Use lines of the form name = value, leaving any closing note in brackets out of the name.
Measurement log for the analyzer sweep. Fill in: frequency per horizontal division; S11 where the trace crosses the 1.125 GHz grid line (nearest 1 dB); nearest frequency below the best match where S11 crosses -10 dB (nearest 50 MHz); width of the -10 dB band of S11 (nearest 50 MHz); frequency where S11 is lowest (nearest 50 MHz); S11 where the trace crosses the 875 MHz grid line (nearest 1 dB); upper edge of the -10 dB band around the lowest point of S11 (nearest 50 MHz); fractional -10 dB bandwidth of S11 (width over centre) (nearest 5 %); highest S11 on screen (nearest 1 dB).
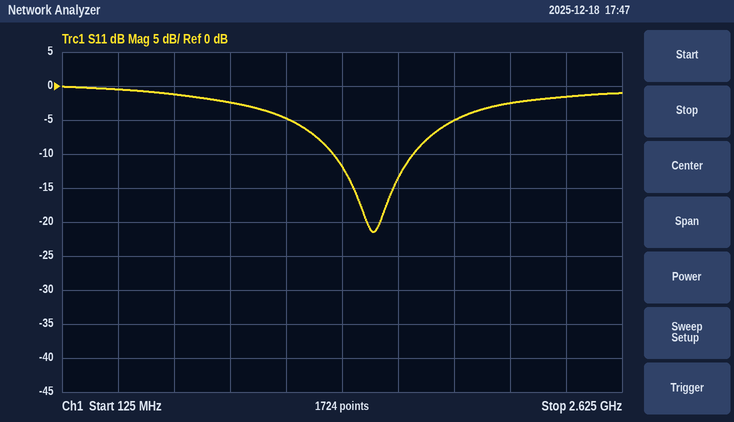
frequency per horizontal division = 250 MHz
S11 where the trace crosses the 1.125 GHz grid line = -5 dB
nearest frequency below the best match where S11 crosses -10 dB = 1.35 GHz
width of the -10 dB band of S11 = 350 MHz
frequency where S11 is lowest = 1.50 GHz
S11 where the trace crosses the 875 MHz grid line = -2 dB
upper edge of the -10 dB band around the lowest point of S11 = 1.70 GHz
fractional -10 dB bandwidth of S11 (width over centre) = 25 %
highest S11 on screen = 0 dB
